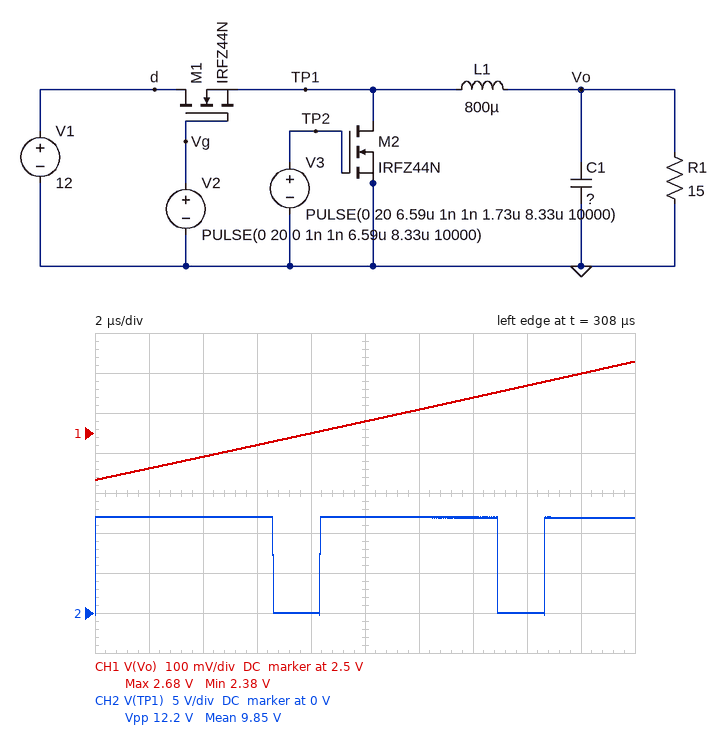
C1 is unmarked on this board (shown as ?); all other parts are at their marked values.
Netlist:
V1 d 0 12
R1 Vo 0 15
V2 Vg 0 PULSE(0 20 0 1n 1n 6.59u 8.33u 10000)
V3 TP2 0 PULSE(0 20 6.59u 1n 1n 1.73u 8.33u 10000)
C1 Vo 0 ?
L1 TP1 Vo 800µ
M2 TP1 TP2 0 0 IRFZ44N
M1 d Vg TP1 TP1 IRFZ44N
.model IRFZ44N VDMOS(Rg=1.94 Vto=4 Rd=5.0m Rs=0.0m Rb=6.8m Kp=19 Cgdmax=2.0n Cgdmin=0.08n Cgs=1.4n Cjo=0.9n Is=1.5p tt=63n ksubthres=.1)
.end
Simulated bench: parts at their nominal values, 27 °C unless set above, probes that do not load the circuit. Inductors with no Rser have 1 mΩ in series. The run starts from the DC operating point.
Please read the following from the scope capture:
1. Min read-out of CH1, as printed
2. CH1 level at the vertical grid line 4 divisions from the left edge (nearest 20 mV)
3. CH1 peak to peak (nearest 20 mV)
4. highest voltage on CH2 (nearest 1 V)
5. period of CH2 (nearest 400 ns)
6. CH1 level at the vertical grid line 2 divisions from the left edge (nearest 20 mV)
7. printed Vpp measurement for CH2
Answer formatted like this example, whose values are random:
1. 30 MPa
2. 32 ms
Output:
1. 2.38 V
2. 2.50 V
3. 300 mV
4. 12 V
5. 8.4 µs
6. 2.44 V
7. 12.2 V
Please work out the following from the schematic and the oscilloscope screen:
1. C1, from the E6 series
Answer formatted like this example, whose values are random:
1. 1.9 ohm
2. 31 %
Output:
1. 220 µF
